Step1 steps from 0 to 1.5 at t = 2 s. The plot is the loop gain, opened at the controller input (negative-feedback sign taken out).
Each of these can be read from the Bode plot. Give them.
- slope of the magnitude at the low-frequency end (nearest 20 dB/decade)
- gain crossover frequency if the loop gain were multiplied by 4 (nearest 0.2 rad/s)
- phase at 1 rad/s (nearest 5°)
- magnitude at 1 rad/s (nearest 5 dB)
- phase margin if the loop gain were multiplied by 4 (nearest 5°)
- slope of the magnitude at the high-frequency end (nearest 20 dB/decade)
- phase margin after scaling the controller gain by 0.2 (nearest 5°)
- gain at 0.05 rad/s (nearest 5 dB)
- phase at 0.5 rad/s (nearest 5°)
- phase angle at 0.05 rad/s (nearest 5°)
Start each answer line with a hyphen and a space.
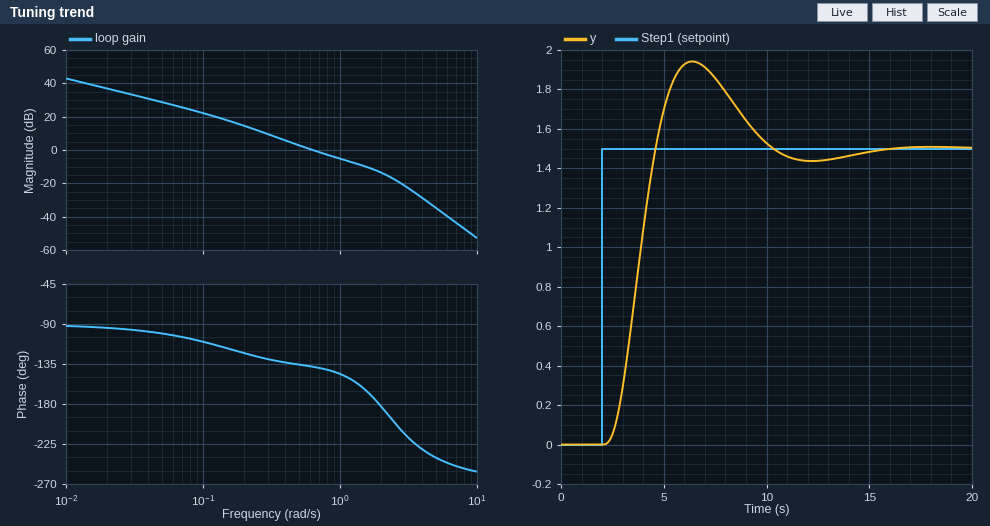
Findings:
- -20 dB/decade
- 1.8 rad/s
- -145°
- -5 dB
- 5°
- -60 dB/decade
- 55°
- 30 dB
- -135°
- -100°
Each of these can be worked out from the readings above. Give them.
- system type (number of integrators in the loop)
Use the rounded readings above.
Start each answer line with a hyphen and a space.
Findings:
- 1
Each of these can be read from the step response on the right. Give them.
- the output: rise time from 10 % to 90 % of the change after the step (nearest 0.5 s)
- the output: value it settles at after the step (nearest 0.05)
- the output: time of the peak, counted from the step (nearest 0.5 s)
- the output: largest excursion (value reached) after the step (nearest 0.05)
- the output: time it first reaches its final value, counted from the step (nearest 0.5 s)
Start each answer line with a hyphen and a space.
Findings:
- 1.5 s
- 1.50
- 4.5 s
- 1.95
- 2.5 s
